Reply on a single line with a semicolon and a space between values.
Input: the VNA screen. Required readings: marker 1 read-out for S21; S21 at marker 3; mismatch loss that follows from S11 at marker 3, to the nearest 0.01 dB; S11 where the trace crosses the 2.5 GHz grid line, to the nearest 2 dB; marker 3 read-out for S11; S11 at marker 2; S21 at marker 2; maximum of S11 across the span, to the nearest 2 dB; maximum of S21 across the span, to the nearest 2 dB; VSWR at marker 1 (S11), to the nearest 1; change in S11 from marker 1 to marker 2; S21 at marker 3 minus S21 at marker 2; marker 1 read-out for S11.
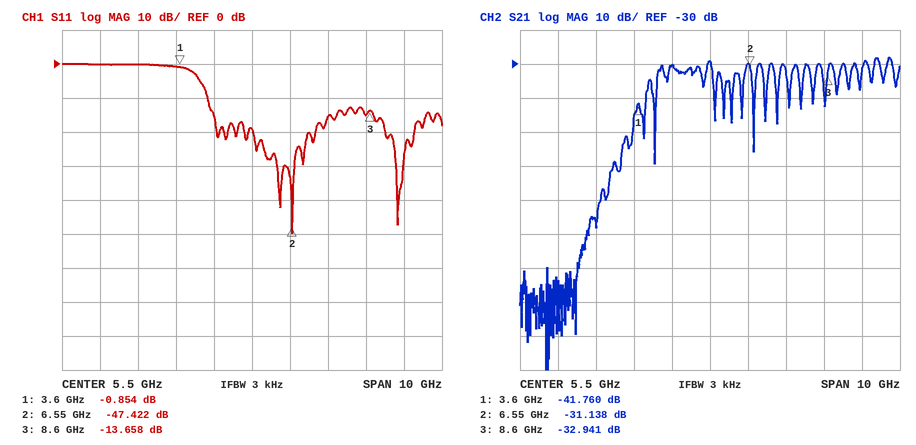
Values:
-41.760 dB; -32.941 dB; 0.19 dB; 0 dB; -13.658 dB; -47.422 dB; -31.138 dB; 0 dB; -28 dB; 20; -46.568 dB; -1.803 dB; -0.854 dB
